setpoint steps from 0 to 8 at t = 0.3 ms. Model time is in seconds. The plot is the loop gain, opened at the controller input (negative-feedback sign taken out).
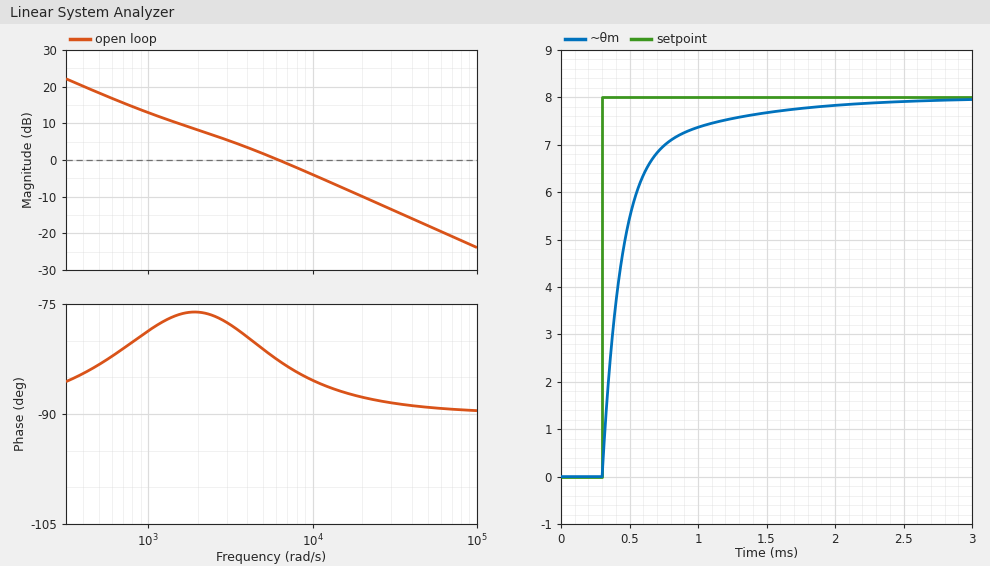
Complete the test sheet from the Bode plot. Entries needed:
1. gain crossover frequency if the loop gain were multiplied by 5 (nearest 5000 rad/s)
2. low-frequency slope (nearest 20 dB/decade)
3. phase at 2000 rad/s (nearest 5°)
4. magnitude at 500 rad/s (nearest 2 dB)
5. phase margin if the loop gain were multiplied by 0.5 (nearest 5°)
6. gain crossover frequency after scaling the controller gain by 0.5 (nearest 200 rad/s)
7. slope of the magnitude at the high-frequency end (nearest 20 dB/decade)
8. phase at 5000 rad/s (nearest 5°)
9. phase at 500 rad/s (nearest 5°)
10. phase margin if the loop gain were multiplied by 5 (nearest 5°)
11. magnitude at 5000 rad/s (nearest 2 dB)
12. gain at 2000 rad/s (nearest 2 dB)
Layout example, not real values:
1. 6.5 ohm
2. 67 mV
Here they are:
1. 30000 rad/s
2. -20 dB/decade
3. -75°
4. 18 dB
5. 105°
6. 2800 rad/s
7. -20 dB/decade
8. -80°
9. -85°
10. 90°
11. 2 dB
12. 8 dB
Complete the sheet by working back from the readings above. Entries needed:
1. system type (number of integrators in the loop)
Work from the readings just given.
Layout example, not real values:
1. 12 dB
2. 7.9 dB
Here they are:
1. 1
